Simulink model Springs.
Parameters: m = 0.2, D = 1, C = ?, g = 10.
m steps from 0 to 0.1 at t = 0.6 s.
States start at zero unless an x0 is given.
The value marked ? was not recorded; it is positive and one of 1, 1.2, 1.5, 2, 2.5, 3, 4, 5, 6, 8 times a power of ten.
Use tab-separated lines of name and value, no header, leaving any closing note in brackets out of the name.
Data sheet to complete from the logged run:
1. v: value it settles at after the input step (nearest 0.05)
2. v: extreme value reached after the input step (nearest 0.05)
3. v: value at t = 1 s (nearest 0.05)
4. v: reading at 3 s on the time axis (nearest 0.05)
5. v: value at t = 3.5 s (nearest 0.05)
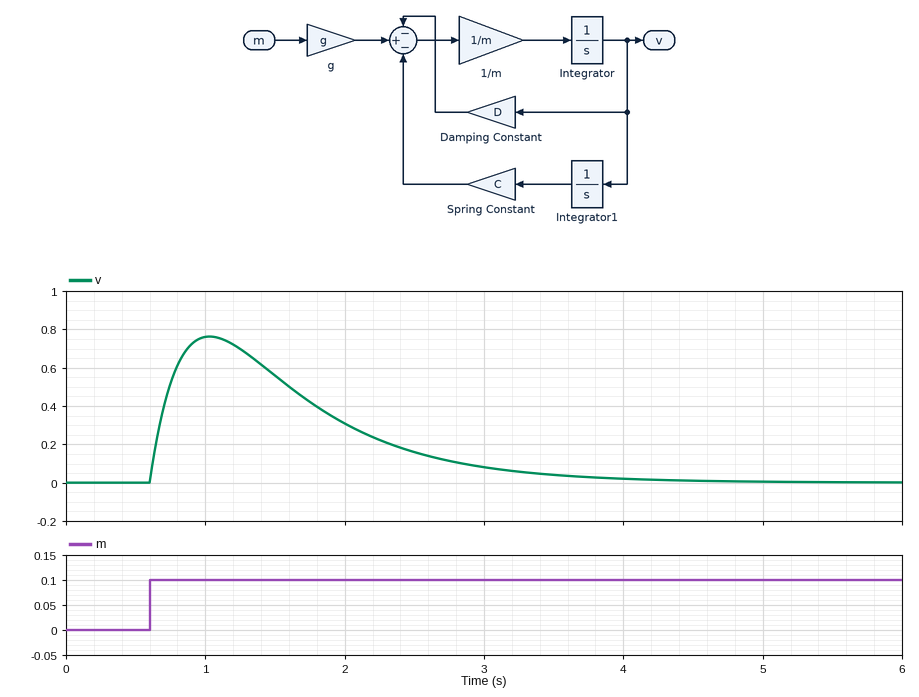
v: value it settles at after the input step	0.00
v: extreme value reached after the input step	0.75
v: value at t = 1 s	0.75
v: reading at 3 s on the time axis	0.10
v: value at t = 3.5 s	0.05
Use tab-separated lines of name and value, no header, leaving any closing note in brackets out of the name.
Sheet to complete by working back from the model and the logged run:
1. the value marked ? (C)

the value marked ?	1
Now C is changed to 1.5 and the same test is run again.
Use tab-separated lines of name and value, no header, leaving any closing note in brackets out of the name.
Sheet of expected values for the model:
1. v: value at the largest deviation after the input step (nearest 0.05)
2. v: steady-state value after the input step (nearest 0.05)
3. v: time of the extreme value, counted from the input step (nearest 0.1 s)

v: value at the largest deviation after the input step	0.70
v: steady-state value after the input step	0.00
v: time of the extreme value, counted from the input step	0.4 s
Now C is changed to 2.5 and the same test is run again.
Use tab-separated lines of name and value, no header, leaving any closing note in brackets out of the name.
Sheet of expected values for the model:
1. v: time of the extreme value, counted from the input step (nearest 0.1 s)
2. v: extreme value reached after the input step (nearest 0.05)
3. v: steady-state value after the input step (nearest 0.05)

v: time of the extreme value, counted from the input step	0.3 s
v: extreme value reached after the input step	0.65
v: steady-state value after the input step	0.00
